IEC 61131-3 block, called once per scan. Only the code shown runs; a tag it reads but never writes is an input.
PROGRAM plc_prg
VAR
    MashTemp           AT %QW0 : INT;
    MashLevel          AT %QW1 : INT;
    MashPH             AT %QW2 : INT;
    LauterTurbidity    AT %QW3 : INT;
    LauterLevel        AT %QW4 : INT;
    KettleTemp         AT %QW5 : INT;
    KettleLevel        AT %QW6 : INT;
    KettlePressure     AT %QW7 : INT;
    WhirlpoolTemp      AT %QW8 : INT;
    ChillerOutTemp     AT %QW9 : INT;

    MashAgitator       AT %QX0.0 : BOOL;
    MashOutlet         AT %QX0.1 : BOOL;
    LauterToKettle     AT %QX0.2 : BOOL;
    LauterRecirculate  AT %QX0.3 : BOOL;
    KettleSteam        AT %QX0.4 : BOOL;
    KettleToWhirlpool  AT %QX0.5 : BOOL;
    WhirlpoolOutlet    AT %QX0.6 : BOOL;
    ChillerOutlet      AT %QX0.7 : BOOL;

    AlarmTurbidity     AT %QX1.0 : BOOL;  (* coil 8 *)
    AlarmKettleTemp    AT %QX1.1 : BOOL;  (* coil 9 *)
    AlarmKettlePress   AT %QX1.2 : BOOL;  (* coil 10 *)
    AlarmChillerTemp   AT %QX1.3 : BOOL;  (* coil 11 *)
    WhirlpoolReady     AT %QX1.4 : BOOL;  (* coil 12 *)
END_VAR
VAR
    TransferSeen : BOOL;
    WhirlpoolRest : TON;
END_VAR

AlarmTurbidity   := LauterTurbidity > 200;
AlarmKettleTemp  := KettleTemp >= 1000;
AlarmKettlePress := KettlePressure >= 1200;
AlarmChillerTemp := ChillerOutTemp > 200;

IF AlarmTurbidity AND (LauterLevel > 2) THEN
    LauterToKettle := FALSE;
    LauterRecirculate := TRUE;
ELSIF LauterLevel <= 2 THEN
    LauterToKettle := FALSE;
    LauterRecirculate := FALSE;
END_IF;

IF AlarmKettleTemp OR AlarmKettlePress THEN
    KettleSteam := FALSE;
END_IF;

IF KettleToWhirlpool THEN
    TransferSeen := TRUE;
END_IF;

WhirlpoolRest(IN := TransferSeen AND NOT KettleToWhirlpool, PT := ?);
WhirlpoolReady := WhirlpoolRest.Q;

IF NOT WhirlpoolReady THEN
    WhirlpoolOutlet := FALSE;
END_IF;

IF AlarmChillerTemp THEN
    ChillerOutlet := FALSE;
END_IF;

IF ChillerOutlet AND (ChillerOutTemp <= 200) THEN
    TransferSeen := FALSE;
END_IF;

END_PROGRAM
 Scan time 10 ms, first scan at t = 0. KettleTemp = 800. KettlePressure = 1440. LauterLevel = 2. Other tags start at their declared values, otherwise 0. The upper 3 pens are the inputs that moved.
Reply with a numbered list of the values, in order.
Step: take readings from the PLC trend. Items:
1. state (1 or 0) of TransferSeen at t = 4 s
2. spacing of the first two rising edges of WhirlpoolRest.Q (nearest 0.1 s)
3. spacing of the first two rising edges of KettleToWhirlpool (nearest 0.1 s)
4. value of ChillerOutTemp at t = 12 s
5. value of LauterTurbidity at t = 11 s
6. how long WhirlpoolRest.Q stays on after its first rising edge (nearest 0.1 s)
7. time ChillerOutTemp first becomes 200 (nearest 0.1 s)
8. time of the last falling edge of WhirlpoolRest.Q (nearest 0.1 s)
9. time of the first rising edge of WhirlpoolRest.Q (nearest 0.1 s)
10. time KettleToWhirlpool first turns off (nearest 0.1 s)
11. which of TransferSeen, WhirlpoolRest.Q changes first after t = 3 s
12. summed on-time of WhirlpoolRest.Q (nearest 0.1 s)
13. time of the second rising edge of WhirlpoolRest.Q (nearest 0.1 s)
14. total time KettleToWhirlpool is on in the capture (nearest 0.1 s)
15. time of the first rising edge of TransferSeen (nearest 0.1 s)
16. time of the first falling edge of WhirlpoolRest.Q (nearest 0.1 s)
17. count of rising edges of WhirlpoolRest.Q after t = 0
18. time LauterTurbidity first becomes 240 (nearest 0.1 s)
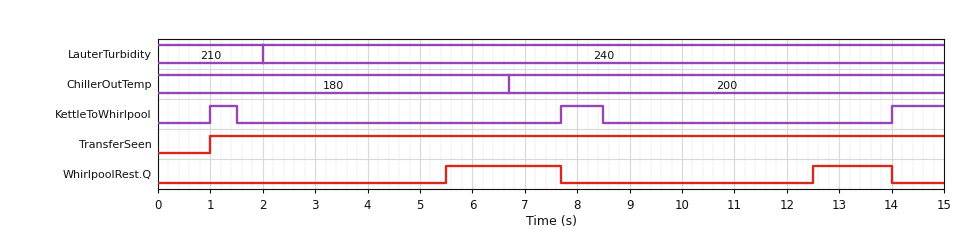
1. 1
2. 7.0 s
3. 6.7 s
4. 200
5. 240
6. 2.2 s
7. 6.7 s
8. 14.0 s
9. 5.5 s
10. 1.5 s
11. WhirlpoolRest.Q
12. 3.7 s
13. 12.5 s
14. 2.3 s
15. 1.0 s
16. 7.7 s
17. 2
18. 2.0 s
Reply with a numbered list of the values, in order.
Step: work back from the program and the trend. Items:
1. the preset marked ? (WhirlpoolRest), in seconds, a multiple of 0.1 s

1. 4.0 s
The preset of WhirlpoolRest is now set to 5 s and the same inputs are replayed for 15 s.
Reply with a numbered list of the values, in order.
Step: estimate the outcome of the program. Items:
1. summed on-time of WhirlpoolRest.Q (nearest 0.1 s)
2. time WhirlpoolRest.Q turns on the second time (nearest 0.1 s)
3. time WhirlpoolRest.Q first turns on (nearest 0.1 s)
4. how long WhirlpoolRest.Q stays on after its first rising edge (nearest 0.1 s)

1. 1.7 s
2. 13.5 s
3. 6.5 s
4. 1.2 s
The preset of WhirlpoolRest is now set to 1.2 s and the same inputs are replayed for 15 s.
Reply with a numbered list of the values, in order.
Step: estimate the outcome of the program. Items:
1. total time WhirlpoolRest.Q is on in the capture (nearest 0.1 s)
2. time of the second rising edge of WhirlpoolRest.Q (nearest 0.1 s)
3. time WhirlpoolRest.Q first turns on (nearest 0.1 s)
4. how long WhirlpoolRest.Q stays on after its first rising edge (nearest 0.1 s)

1. 9.3 s
2. 9.7 s
3. 2.7 s
4. 5.0 s
